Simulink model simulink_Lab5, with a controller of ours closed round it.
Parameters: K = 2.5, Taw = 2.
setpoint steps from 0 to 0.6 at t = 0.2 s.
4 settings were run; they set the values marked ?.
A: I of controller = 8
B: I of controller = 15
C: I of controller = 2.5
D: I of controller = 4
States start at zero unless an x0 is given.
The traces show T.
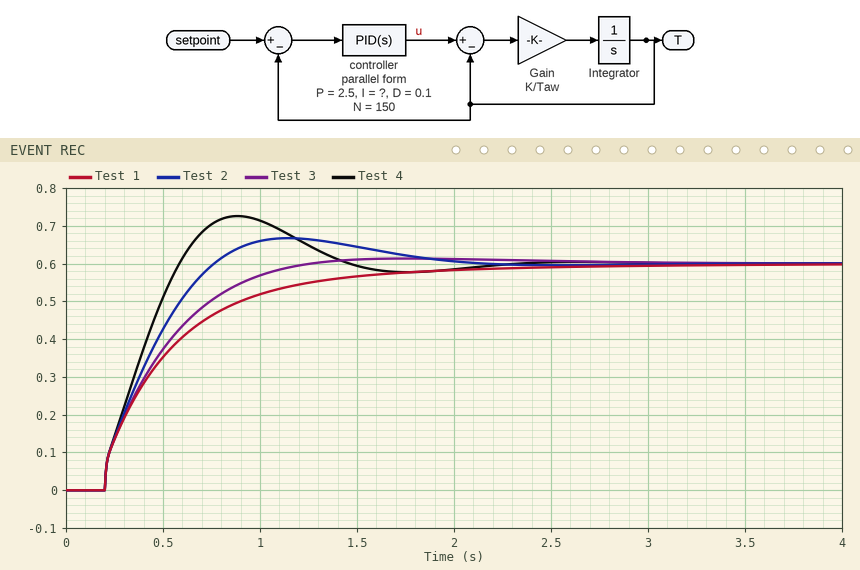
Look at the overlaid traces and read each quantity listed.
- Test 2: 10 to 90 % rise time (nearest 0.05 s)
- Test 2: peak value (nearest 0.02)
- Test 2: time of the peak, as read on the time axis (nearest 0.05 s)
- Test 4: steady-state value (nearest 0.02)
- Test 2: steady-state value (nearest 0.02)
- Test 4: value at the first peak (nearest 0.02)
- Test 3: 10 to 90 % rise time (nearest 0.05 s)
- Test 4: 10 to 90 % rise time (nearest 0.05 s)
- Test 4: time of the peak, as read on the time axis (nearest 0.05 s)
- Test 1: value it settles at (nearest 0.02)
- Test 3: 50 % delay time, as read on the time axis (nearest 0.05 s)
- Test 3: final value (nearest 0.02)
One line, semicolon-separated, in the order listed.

0.45 s; 0.66; 1.15 s; 0.60; 0.60; 0.72; 0.65 s; 0.30 s; 0.90 s; 0.60; 0.40 s; 0.60
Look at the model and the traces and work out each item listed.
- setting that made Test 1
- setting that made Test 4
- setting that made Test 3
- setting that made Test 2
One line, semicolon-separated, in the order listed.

C; B; D; A
